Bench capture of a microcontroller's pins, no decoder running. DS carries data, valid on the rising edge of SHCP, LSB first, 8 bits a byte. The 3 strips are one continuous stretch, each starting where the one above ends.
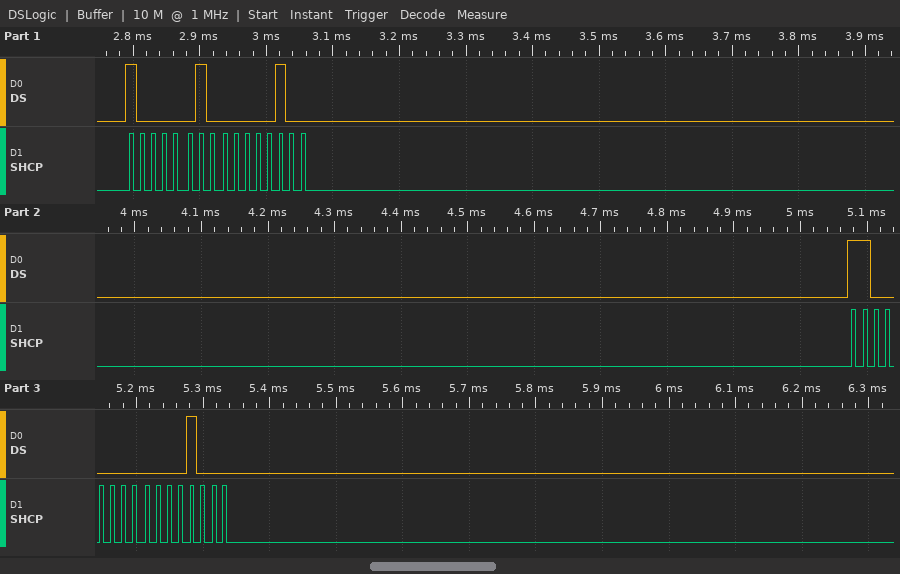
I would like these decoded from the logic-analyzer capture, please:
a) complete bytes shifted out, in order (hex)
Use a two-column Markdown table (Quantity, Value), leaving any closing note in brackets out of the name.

| Quantity | Value |
|---|---|
| complete bytes shifted out, in order | 41 20 03 10 |
